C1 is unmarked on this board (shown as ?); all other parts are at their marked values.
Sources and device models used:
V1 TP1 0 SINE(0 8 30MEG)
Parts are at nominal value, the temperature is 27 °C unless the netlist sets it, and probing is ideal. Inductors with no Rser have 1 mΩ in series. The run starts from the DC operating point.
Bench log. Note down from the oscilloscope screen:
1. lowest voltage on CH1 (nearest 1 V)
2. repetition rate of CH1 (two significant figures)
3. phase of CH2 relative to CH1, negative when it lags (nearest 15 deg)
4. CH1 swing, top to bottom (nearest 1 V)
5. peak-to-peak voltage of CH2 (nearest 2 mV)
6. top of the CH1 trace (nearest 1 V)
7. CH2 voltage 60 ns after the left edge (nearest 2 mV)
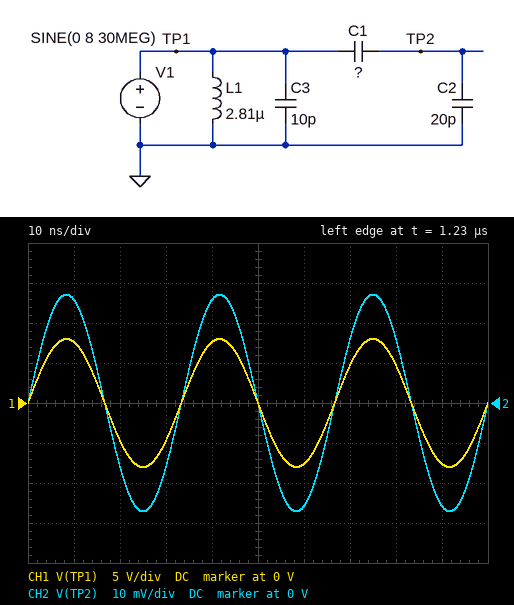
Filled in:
-8 V
30 MHz
0 deg
16 V
54 mV
8 V
-26 mV
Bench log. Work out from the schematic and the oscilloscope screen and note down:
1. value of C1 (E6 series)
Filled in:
68 fF
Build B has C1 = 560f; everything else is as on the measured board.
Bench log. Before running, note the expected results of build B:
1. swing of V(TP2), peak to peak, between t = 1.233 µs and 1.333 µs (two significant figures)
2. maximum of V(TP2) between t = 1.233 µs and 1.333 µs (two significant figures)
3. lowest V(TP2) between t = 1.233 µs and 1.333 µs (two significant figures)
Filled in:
440 mV
220 mV
-220 mV
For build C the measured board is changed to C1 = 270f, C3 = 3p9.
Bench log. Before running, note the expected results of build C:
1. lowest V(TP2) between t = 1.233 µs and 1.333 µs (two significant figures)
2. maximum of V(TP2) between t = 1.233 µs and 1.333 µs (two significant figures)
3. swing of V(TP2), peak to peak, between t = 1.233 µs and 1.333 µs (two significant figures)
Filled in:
-110 mV
110 mV
210 mV
